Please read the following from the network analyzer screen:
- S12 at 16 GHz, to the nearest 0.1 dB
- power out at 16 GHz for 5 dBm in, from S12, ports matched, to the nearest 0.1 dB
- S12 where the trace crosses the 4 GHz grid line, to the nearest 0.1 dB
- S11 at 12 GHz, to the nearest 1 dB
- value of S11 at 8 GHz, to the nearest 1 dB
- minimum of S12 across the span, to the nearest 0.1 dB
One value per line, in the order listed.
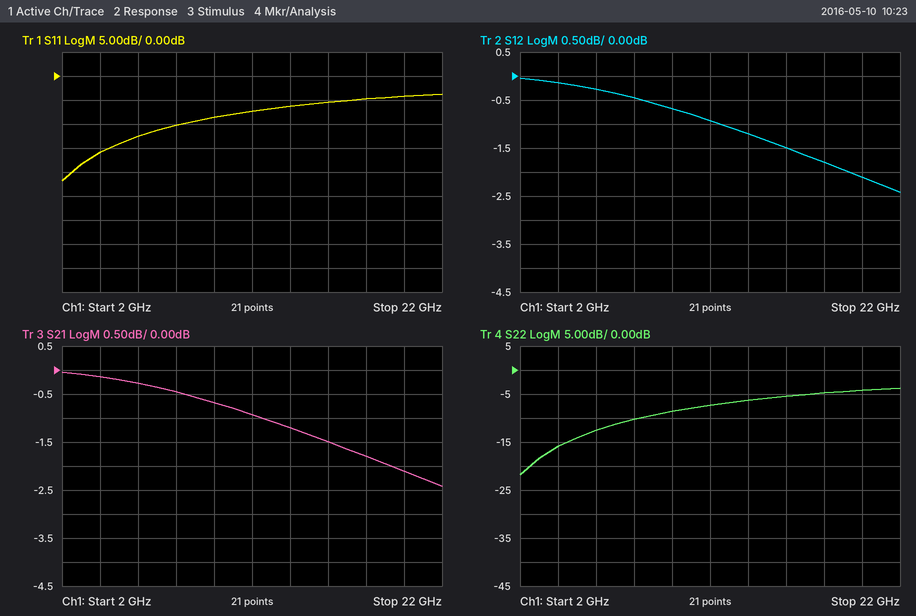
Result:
-1.5 dB
3.5 dBm
-0.1 dB
-7 dB
-10 dB
-2.4 dB
